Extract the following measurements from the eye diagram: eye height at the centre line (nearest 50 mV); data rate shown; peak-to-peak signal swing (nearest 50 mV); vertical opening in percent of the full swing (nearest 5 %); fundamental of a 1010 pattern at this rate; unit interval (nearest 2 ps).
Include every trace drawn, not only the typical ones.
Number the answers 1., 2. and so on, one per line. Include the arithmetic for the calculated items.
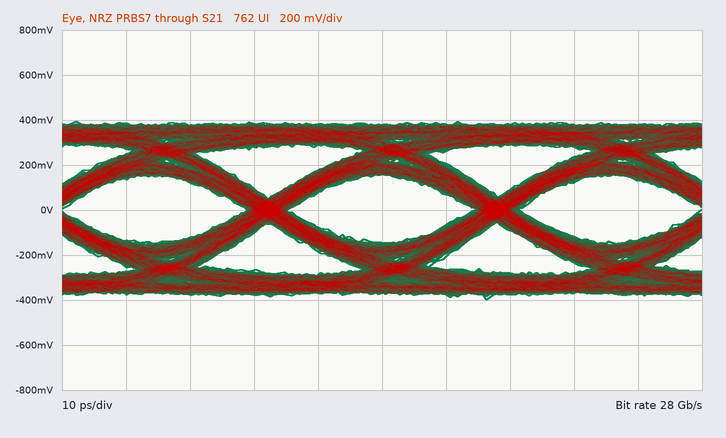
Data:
1. 300 mV
2. 28 Gb/s
3. 800 mV
4. 300 mV / 800 mV ≈ 37.5 %, so 40 % to the nearest 5 %
5. 14 GHz
6. 36 ps
